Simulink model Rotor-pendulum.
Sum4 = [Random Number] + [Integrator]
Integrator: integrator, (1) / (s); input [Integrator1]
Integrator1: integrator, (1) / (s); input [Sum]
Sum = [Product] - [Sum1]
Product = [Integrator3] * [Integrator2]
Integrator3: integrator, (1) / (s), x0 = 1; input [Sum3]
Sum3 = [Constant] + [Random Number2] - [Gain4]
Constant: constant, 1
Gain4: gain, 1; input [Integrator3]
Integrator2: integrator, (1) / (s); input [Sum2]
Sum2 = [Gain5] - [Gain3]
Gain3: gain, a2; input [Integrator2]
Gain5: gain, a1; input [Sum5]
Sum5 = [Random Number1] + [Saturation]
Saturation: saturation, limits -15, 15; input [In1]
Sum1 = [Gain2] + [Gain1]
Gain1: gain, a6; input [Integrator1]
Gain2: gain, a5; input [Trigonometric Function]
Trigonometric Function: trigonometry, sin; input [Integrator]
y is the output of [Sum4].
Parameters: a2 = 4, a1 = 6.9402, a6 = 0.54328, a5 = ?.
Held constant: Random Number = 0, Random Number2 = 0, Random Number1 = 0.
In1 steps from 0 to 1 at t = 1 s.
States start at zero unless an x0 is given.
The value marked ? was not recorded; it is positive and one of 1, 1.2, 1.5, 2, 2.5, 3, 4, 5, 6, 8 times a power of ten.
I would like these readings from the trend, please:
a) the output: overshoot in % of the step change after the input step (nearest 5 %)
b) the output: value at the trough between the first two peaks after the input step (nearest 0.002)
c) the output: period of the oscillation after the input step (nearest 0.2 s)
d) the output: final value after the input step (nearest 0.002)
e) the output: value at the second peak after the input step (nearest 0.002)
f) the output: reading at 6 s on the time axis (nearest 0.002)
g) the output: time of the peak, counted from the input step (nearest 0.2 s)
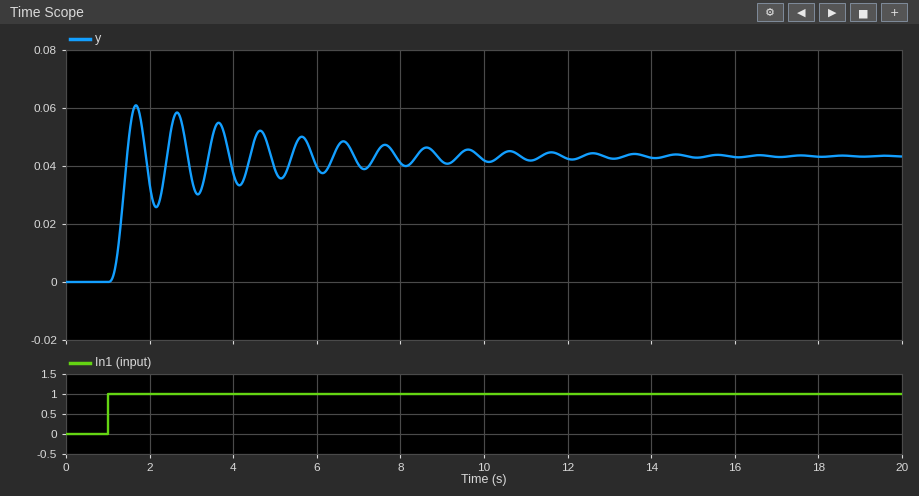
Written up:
40 %
0.026
1.0 s
0.044
0.058
0.040
0.6 s
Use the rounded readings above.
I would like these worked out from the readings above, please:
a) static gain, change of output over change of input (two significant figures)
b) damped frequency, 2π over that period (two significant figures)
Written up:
0.044
6.3 rad/s
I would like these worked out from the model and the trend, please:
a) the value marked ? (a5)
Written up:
40
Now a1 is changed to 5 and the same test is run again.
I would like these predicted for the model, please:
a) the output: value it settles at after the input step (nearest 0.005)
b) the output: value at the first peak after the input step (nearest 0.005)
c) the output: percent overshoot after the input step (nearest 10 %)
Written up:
0.030
0.045
40 %
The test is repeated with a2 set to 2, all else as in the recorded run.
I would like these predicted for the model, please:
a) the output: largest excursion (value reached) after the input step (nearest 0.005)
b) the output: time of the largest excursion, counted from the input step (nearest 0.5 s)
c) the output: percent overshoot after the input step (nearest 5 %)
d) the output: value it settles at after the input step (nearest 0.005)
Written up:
0.100
1.5 s
15 %
0.085
